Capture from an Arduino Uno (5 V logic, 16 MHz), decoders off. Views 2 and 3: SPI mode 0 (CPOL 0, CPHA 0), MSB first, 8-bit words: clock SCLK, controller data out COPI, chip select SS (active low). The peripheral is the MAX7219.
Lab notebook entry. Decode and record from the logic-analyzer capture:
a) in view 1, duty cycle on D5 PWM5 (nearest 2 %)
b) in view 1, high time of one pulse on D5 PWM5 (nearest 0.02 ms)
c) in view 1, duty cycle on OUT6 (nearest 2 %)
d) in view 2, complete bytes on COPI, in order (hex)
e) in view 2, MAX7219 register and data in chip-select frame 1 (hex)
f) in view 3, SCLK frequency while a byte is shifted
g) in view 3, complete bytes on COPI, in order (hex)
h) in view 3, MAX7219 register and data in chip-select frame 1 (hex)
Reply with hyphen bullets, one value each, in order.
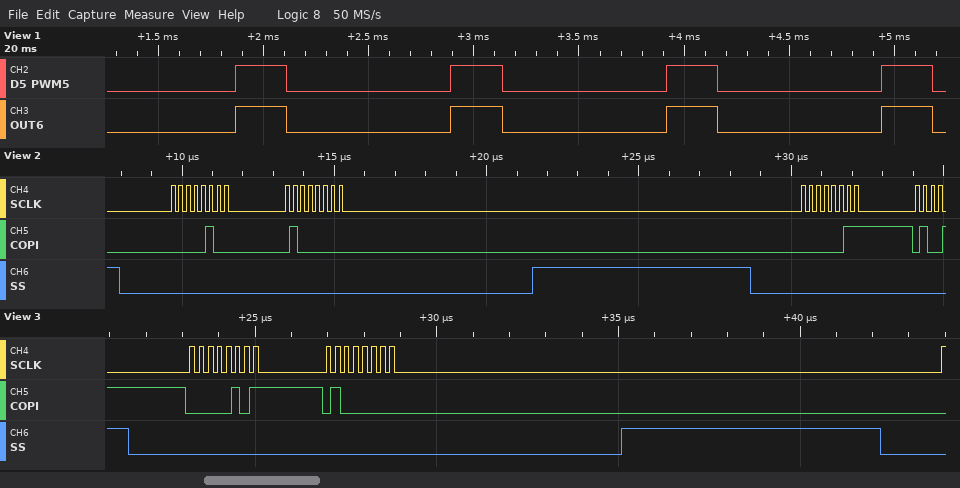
- 24 %
- 0.24 ms
- 24 %
- 04 40 03
- register 0x4, data 0x40
- 4 MHz
- 05 40
- register 0x5, data 0x40
